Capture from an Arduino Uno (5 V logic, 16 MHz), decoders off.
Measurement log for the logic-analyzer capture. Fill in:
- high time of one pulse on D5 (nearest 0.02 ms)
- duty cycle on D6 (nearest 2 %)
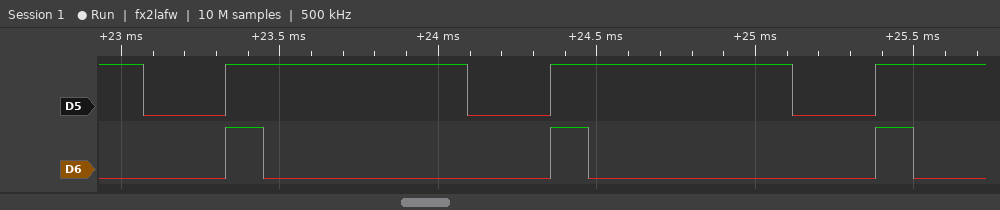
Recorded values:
0.76 ms
12 %
